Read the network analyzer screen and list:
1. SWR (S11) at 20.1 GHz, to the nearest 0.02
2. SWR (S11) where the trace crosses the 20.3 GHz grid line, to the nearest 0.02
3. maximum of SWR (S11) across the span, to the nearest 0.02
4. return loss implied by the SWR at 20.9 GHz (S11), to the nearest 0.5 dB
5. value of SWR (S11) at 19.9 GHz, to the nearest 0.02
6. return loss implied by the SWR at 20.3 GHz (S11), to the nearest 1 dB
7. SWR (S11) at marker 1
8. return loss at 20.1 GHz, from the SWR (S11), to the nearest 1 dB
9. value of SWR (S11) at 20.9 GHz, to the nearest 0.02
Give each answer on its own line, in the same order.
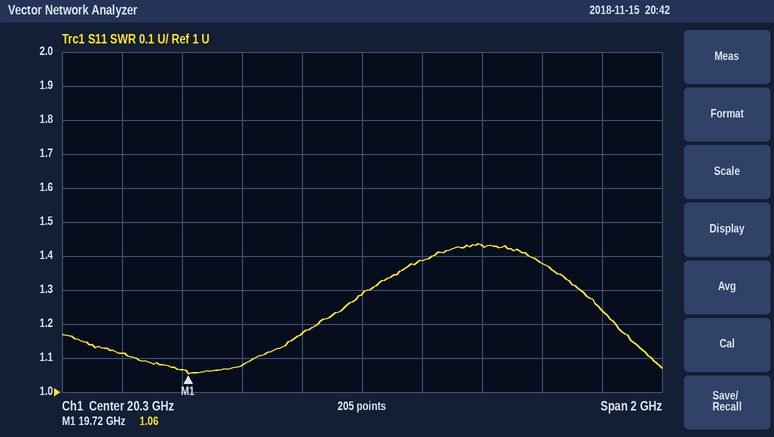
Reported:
1.18
1.28
1.44
16.0 dB
1.08
18 dB
1.06
22 dB
1.38
